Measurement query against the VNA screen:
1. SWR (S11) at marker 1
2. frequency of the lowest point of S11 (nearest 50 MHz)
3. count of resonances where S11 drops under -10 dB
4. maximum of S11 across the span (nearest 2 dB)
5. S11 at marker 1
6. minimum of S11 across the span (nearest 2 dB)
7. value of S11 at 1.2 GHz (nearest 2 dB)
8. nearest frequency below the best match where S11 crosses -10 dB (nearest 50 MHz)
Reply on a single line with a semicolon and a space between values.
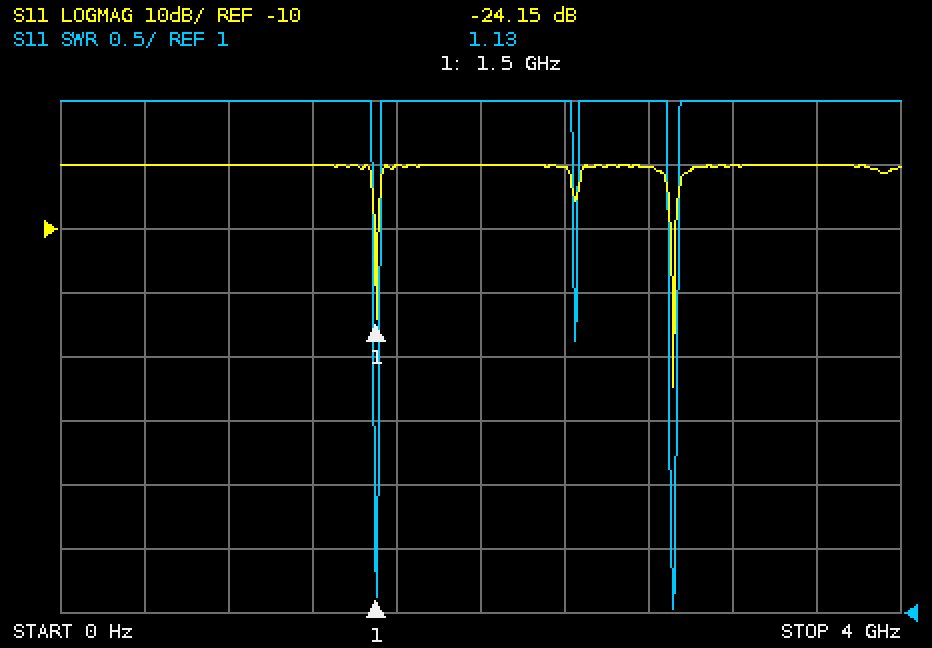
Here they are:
1.13; 2.90 GHz; 2; 0 dB; -24.15 dB; -34 dB; 0 dB; 2.90 GHz
